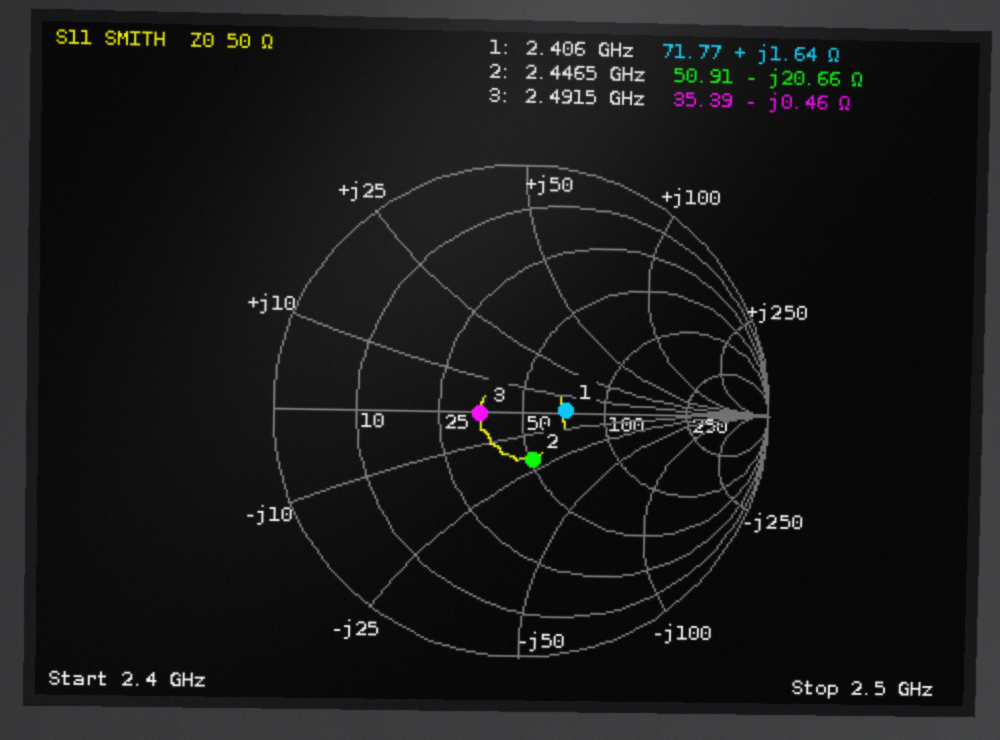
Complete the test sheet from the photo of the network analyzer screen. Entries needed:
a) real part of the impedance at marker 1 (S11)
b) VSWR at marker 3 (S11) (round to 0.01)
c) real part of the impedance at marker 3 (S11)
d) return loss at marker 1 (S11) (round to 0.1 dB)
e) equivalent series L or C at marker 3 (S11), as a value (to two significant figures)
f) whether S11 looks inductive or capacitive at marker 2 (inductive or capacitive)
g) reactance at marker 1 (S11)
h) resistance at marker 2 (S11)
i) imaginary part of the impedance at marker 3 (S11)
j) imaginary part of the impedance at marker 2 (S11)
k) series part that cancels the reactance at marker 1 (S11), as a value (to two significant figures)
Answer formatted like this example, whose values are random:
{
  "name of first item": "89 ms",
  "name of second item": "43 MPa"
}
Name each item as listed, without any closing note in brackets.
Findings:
{
  "real part of the impedance at marker 1": "71.77 Ω",
  "VSWR at marker 3 (S11)": "1.41",
  "real part of the impedance at marker 3": "35.39 Ω",
  "return loss at marker 1 (S11)": "14.9 dB",
  "equivalent series L or C at marker 3 (S11), as a value": "140 pF",
  "whether S11 looks inductive or capacitive at marker 2": "capacitive",
  "reactance at marker 1": "+1.64 Ω",
  "resistance at marker 2": "50.91 Ω",
  "imaginary part of the impedance at marker 3": "-0.46 Ω",
  "imaginary part of the impedance at marker 2": "-20.66 Ω",
  "series part that cancels the reactance at marker 1 (S11), as a value": "40 pF"
}
